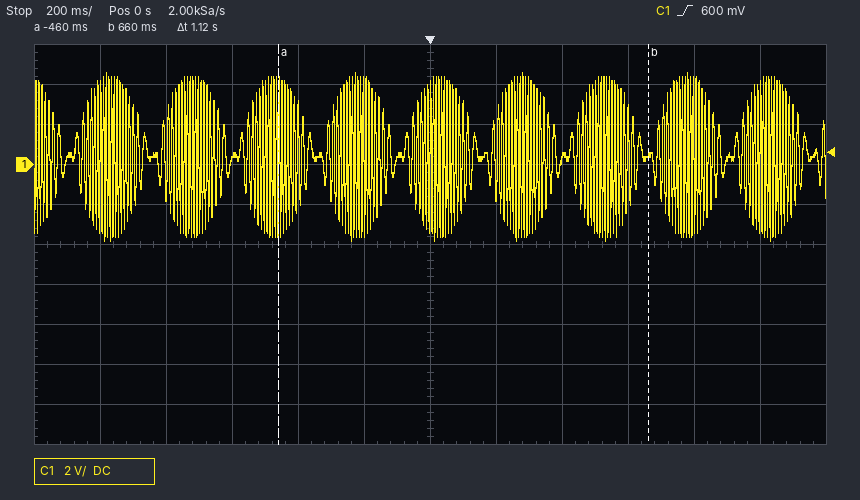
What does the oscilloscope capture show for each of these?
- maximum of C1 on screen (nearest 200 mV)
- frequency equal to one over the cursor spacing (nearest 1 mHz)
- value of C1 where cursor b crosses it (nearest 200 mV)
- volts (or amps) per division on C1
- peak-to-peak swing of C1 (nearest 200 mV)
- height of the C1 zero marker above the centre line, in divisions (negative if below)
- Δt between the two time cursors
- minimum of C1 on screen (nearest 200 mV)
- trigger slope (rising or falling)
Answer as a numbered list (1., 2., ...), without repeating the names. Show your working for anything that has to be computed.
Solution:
1. 4.6 V
2. 1 / 1.12 s ≈ 893 mHz
3. 400 mV
4. 2 V
5. 4.6 V − (-3.8 V) = 8.4 V
6. +2.0 div
7. 1.12 s
8. -3.8 V
9. rising
